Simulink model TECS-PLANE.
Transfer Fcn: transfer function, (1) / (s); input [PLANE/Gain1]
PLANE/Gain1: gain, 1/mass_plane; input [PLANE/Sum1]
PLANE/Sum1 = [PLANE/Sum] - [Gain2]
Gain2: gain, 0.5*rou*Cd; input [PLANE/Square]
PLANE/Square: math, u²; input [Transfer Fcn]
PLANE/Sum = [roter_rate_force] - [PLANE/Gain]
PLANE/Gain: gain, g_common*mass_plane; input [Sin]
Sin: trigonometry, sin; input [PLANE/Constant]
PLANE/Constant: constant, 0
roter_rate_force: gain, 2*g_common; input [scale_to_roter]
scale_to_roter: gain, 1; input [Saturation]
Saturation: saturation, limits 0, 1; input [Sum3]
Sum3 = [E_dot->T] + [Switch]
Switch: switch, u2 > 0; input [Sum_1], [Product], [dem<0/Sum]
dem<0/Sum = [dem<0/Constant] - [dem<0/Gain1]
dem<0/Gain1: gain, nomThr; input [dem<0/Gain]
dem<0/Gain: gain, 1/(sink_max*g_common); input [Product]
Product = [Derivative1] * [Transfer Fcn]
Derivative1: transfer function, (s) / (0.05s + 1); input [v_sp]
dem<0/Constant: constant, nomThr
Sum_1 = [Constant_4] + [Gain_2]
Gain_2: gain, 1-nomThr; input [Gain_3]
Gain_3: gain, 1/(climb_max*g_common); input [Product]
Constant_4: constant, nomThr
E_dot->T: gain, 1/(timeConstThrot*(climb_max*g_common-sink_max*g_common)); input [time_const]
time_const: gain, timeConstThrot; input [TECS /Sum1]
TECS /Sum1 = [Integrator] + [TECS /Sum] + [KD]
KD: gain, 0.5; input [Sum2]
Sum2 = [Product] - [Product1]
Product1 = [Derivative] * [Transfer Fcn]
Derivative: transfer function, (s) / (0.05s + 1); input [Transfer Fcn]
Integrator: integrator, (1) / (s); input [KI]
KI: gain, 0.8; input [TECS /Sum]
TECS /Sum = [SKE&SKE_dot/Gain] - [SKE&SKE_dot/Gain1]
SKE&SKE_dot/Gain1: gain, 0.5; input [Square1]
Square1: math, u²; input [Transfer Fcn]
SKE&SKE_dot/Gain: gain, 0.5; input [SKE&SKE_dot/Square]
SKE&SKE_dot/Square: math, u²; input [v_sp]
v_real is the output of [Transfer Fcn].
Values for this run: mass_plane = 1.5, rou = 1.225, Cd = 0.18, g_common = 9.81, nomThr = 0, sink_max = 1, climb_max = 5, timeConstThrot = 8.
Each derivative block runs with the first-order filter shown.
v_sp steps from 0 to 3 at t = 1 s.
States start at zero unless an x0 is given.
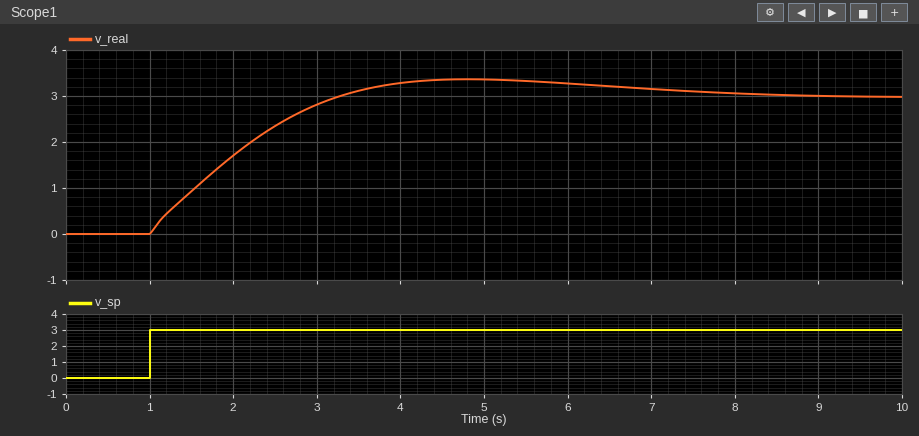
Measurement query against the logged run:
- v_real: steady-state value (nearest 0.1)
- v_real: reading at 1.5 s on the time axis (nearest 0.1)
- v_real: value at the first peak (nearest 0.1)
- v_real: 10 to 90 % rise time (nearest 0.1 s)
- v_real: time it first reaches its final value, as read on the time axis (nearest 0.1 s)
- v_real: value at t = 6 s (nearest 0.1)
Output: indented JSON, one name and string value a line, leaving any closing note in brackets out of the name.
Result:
{
  "v_real: steady-state value": "3.0",
  "v_real: reading at 1.5 s on the time axis": "0.9",
  "v_real: value at the first peak": "3.4",
  "v_real: 10 to 90 % rise time": "1.7 s",
  "v_real: time it first reaches its final value, as read on the time axis": "3.3 s",
  "v_real: value at t = 6 s": "3.3"
}
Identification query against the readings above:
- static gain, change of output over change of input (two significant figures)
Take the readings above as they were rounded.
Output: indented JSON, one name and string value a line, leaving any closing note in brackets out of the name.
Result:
{
  "static gain, change of output over change of input": "1.0"
}
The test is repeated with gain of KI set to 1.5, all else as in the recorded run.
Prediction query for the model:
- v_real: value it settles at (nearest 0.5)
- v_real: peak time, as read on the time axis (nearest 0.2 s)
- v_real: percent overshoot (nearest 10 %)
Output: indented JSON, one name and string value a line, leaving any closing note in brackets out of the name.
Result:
{
  "v_real: value it settles at": "3.0",
  "v_real: peak time, as read on the time axis": "3.8 s",
  "v_real: percent overshoot": "20 %"
}
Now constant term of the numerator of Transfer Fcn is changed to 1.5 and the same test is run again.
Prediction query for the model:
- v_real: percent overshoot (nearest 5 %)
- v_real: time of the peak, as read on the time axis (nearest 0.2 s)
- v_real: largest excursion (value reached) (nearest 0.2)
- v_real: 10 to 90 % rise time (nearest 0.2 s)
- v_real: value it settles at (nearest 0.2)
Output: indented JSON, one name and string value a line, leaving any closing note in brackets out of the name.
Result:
{
  "v_real: percent overshoot": "10 %",
  "v_real: time of the peak, as read on the time axis": "4.4 s",
  "v_real: largest excursion (value reached)": "3.2",
  "v_real: 10 to 90 % rise time": "1.4 s",
  "v_real: value it settles at": "3.0"
}
